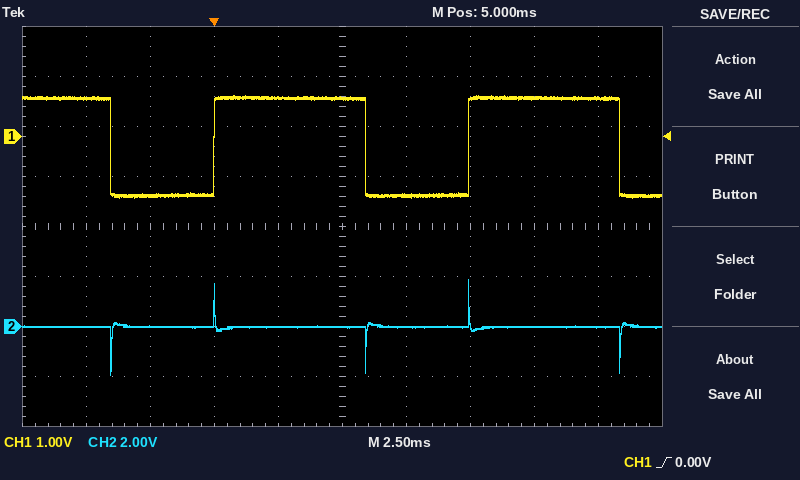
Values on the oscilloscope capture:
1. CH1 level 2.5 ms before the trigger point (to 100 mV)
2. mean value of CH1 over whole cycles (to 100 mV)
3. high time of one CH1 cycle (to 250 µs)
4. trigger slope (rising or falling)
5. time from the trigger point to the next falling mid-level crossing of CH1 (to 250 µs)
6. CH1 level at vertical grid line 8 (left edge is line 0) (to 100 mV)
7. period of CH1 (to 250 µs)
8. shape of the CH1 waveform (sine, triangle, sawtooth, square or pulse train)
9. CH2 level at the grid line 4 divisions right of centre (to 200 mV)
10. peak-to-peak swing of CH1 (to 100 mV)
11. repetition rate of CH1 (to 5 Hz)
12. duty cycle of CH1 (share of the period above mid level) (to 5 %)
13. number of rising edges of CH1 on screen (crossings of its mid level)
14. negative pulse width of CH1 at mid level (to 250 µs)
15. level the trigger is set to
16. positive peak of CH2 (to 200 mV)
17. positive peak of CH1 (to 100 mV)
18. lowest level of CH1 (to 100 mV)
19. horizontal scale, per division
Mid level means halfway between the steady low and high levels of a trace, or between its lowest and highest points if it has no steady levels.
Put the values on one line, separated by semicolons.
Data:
-1.2 V; 0.0 V; 6.00 ms; rising; 6.00 ms; 800 mV; 10.00 ms; pulse train; 0.0 V; 2.0 V; 100 Hz; 60 %; 2; 4.00 ms; 0.00 V; 1.8 V; 800 mV; -1.2 V; 2.5 ms
